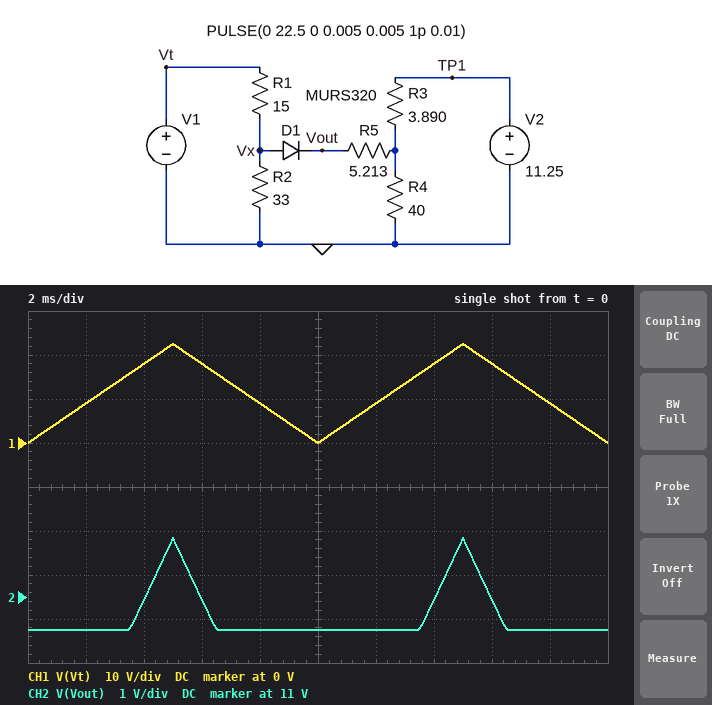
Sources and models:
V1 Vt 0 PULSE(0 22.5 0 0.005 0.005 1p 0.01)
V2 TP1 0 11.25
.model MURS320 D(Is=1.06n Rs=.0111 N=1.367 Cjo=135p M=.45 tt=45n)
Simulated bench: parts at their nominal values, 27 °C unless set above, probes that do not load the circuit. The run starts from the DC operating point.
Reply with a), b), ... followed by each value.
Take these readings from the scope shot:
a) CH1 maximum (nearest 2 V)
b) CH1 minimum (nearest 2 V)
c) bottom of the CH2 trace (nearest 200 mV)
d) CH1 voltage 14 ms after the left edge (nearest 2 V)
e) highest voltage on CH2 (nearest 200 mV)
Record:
a) 22 V
b) 0 V
c) 10.2 V
d) 18 V
e) 12.4 V
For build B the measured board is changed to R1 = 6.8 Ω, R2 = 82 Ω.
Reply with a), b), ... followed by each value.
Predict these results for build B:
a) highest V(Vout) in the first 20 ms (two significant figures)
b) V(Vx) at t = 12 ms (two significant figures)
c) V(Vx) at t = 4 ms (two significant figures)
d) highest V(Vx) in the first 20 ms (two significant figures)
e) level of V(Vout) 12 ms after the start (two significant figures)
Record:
a) 16 V
b) 8.3 V
c) 14 V
d) 17 V
e) 10 V
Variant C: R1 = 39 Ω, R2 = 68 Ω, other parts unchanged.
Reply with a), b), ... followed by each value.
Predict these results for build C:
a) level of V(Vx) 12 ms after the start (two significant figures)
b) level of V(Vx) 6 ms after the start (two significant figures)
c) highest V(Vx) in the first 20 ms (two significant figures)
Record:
a) 5.7 V
b) 11 V
c) 12 V
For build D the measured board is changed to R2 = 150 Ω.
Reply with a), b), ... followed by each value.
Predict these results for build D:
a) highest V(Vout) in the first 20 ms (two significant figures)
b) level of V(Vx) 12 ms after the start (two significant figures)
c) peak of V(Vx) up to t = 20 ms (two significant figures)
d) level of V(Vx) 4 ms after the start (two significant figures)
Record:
a) 14 V
b) 8.2 V
c) 15 V
d) 13 V
